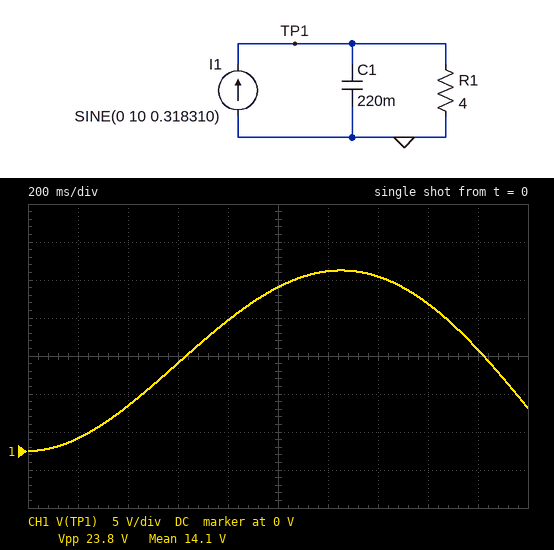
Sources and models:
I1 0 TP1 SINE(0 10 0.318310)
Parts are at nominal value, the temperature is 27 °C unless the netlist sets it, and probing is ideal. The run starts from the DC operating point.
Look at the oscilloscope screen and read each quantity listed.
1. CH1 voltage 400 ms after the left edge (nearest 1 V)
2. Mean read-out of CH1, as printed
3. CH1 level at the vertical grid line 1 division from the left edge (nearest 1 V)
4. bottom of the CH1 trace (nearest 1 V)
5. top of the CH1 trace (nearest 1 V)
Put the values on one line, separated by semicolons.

6 V; 14.1 V; 2 V; 0 V; 24 V
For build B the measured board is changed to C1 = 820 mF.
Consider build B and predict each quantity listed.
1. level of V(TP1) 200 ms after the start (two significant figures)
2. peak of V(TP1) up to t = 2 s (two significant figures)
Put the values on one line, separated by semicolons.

470 mV; 9.8 V
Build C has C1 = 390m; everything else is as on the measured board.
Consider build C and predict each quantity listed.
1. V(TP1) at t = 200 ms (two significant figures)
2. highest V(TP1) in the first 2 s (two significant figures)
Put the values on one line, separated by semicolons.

970 mV; 17 V
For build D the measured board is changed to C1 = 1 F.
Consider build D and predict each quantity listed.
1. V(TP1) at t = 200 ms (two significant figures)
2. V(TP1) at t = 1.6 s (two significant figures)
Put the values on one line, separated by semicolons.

390 mV; 8.2 V
